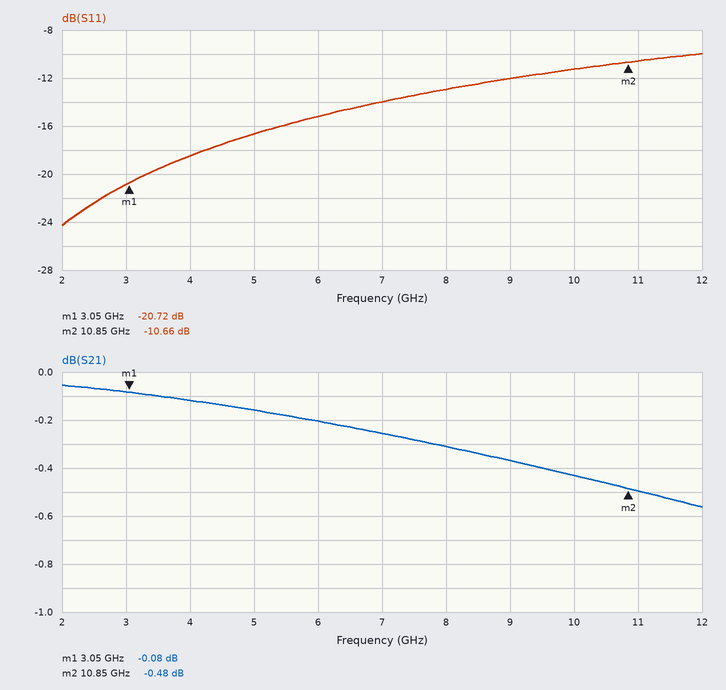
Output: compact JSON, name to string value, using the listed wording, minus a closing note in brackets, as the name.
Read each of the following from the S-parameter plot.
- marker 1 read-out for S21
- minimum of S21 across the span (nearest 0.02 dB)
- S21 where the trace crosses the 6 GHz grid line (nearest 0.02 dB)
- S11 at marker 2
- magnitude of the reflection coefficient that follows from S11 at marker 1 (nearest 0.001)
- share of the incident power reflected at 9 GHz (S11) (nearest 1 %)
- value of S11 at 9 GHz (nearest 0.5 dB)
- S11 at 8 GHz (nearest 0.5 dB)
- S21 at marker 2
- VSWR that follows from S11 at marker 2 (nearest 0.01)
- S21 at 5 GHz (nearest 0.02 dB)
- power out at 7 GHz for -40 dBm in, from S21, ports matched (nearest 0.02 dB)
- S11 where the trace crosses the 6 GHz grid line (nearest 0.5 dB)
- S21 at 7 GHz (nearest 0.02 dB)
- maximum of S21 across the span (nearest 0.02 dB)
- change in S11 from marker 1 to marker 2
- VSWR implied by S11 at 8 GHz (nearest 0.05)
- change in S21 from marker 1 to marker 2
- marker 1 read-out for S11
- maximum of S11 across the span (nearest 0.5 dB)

{"marker 1 read-out for S21": "-0.08 dB", "minimum of S21 across the span": "-0.56 dB", "S21 where the trace crosses the 6 GHz grid line": "-0.20 dB", "S11 at marker 2": "-10.66 dB", "magnitude of the reflection coefficient that follows from S11 at marker 1": "0.092", "share of the incident power reflected at 9 GHz (S11)": "6 %", "value of S11 at 9 GHz": "-12.0 dB", "S11 at 8 GHz": "-13.0 dB", "S21 at marker 2": "-0.48 dB", "VSWR that follows from S11 at marker 2": "1.83", "S21 at 5 GHz": "-0.16 dB", "power out at 7 GHz for -40 dBm in, from S21, ports matched": "-40.26 dBm", "S11 where the trace crosses the 6 GHz grid line": "-15.0 dB", "S21 at 7 GHz": "-0.26 dB", "maximum of S21 across the span": "-0.06 dB", "change in S11 from marker 1 to marker 2": "10.06 dB", "VSWR implied by S11 at 8 GHz": "1.60", "change in S21 from marker 1 to marker 2": "-0.40 dB", "marker 1 read-out for S11": "-20.72 dB", "maximum of S11 across the span": "-10.0 dB"}
